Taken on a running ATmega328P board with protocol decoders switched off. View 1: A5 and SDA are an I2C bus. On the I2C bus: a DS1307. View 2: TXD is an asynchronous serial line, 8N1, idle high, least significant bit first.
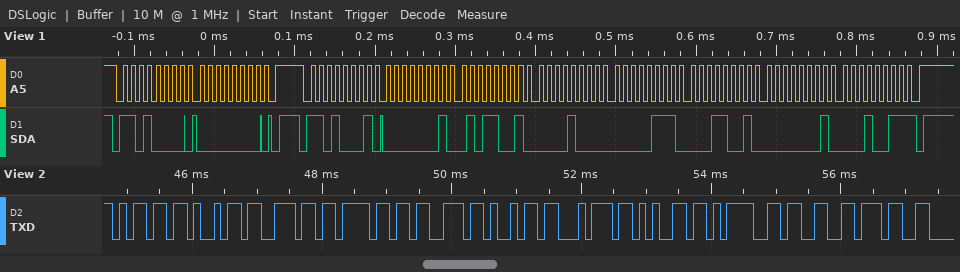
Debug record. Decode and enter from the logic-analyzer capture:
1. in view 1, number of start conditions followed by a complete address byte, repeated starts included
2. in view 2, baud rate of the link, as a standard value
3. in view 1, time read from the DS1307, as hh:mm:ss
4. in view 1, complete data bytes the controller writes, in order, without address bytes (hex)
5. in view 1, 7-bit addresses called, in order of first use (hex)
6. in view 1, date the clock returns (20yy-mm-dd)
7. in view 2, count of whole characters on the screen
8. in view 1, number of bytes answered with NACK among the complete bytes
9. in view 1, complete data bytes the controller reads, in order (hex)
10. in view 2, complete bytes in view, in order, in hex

2
9600 baud
08:59:01
00
0x68
2013-01-19
11
1
01 59 08 07 19 01 13
6D 69 6E 6F 73 69 74 65 3D 33 37
